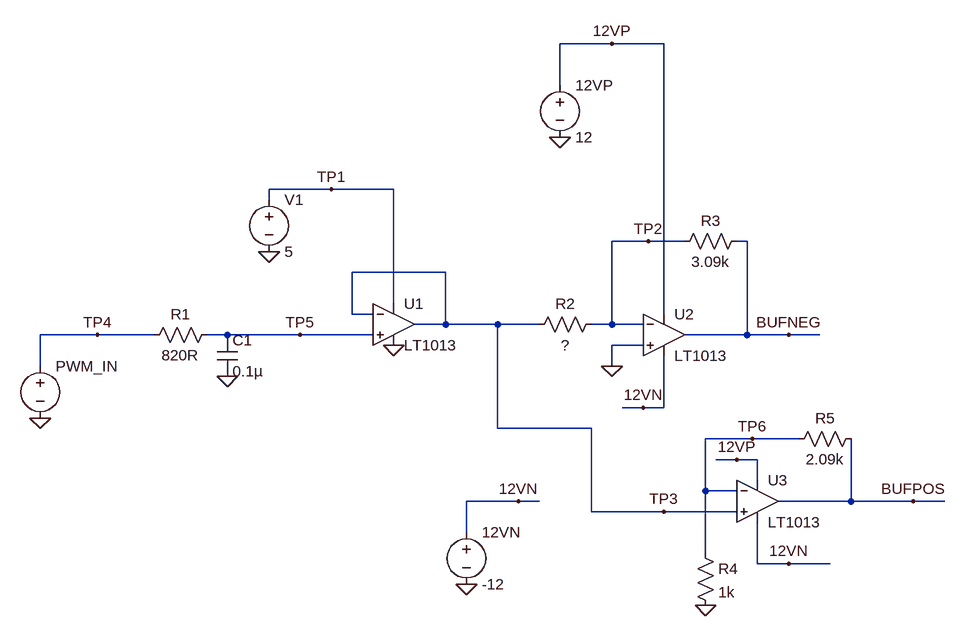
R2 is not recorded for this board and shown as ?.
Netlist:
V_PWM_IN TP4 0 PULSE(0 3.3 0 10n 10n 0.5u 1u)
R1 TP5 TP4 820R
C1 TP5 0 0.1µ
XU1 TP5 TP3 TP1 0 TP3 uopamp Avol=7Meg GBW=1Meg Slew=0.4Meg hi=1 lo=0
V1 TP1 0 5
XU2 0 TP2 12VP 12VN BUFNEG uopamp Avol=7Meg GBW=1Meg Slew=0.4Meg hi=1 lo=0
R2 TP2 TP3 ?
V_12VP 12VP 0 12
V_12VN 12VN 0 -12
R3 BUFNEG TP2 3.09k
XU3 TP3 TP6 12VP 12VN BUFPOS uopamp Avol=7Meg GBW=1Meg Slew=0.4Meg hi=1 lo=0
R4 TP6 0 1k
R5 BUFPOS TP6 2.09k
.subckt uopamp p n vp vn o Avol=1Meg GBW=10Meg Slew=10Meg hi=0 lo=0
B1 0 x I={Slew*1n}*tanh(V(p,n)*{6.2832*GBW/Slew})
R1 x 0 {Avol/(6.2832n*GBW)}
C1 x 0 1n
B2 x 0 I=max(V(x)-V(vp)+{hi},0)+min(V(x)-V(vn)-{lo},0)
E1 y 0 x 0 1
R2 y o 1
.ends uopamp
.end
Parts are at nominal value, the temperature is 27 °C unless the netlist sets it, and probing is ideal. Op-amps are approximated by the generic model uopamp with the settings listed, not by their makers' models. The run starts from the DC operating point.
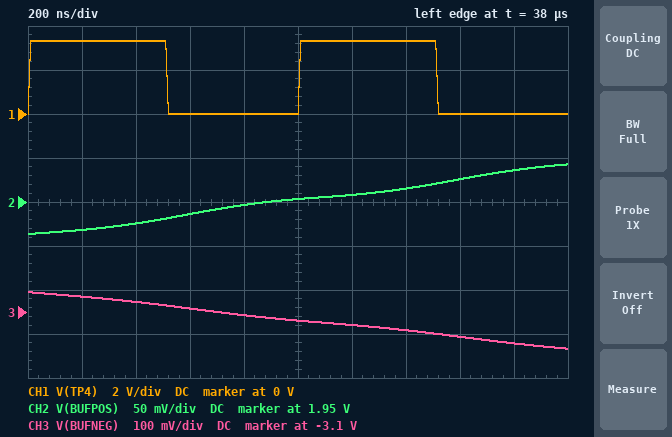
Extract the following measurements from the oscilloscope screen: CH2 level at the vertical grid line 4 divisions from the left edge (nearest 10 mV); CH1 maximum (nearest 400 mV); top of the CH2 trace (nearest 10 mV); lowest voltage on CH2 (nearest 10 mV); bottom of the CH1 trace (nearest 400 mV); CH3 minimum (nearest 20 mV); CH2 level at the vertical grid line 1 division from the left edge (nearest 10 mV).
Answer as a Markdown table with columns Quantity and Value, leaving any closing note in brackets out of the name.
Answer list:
| Quantity | Value |
|---|---|
| CH2 level at the vertical grid line 4 divisions from the left edge | 1.95 V |
| CH1 maximum | 3.2 V |
| top of the CH2 trace | 1.99 V |
| lowest voltage on CH2 | 1.91 V |
| bottom of the CH1 trace | 0 V |
| CH3 minimum | -3.18 V |
| CH2 level at the vertical grid line 1 division from the left edge | 1.92 V |
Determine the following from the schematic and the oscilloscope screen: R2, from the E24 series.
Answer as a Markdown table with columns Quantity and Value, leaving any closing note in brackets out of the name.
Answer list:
| Quantity | Value |
|---|---|
| R2, from the E24 series | 620 Ω |
